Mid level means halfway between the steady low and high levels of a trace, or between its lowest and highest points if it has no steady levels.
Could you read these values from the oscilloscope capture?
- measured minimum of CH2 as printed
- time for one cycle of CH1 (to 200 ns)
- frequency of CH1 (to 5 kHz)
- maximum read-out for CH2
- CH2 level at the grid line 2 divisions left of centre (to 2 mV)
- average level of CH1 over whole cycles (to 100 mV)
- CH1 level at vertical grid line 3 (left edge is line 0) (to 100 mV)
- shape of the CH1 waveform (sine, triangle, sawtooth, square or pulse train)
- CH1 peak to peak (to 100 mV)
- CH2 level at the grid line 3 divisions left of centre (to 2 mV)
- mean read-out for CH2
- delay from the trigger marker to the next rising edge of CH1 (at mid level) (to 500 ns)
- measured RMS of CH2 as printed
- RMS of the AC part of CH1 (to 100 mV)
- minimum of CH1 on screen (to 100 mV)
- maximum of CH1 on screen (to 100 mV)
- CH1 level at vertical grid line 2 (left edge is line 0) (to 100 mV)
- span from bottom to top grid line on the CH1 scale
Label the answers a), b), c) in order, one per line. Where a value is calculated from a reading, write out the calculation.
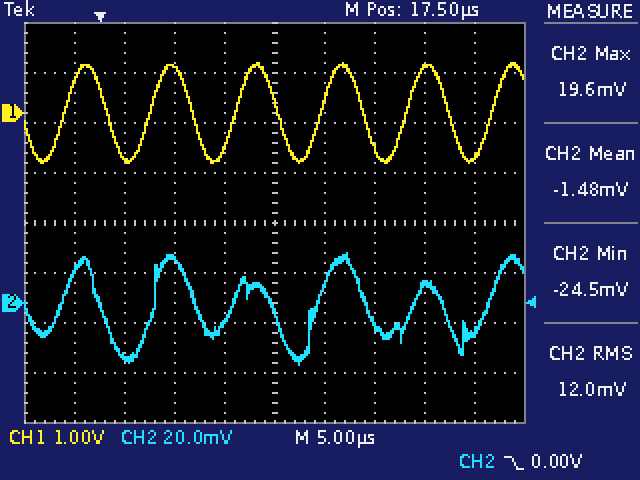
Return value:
a) -24.5 mV
b) 8.6 µs
c) 1 / 8.6 µs ≈ 116 kHz, so 115 kHz to the nearest 5 kHz
d) 19.6 mV
e) 18 mV
f) (1.0 V + (-1.0 V)) / 2 ≈ 0.0 V
g) 900 mV
h) sine
i) 1.0 V − (-1.0 V) = 2.0 V
j) -22 mV
k) -1.48 mV
l) 5.0 µs
m) 12.0 mV
n) 2.0 V / (2√2) ≈ 707 mV, so 700 mV to the nearest 100 mV
o) -1.0 V
p) 1.0 V
q) -900 mV
r) 8 V
